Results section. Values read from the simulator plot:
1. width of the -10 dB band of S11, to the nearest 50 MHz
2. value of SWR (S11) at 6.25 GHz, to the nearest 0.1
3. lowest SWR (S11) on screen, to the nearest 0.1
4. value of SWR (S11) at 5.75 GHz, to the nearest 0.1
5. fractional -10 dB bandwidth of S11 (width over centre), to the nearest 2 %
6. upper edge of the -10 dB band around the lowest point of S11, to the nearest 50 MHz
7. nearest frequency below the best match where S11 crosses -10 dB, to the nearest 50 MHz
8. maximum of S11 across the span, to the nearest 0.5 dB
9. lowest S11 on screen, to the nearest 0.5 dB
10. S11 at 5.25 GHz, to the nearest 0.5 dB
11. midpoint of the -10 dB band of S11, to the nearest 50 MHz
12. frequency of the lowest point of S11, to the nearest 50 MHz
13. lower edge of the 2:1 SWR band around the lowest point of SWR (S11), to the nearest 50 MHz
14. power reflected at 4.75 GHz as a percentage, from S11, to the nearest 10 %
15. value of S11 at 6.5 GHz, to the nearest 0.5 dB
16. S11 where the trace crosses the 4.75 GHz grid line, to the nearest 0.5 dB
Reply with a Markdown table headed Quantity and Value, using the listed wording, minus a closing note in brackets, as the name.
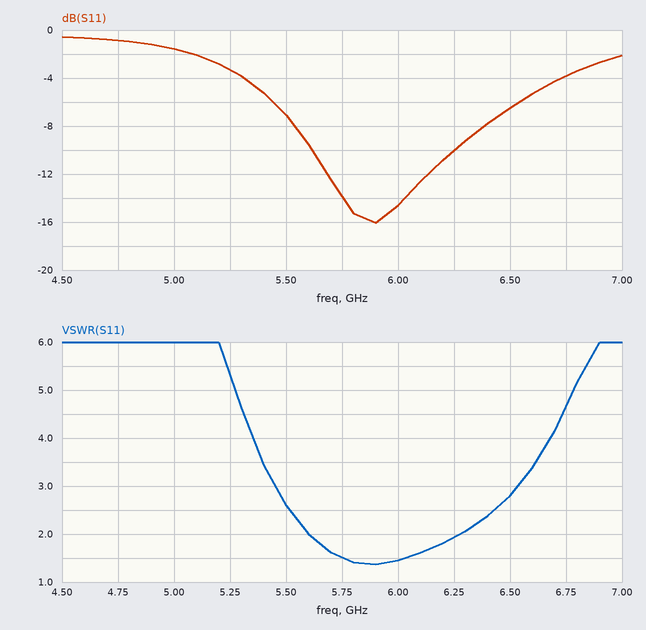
| Quantity | Value |
|---|---|
| width of the -10 dB band of S11, to the nearest 50 MHz | 650 MHz |
| value of SWR (S11) at 6.25 GHz, to the nearest 0.1 | 1.9 |
| lowest SWR (S11) on screen, to the nearest 0.1 | 1.4 |
| value of SWR (S11) at 5.75 GHz, to the nearest 0.1 | 1.5 |
| fractional -10 dB bandwidth of S11 (width over centre), to the nearest 2 % | 10 % |
| upper edge of the -10 dB band around the lowest point of S11, to the nearest 50 MHz | 6.25 GHz |
| nearest frequency below the best match where S11 crosses -10 dB, to the nearest 50 MHz | 5.60 GHz |
| maximum of S11 across the span, to the nearest 0.5 dB | -0.5 dB |
| lowest S11 on screen, to the nearest 0.5 dB | -16.0 dB |
| S11 at 5.25 GHz, to the nearest 0.5 dB | -3.5 dB |
| midpoint of the -10 dB band of S11, to the nearest 50 MHz | 5.95 GHz |
| frequency of the lowest point of S11, to the nearest 50 MHz | 5.90 GHz |
| lower edge of the 2:1 SWR band around the lowest point of SWR (S11), to the nearest 50 MHz | 5.60 GHz |
| power reflected at 4.75 GHz as a percentage, from S11, to the nearest 10 % | 80 % |
| value of S11 at 6.5 GHz, to the nearest 0.5 dB | -6.5 dB |
| S11 where the trace crosses the 4.75 GHz grid line, to the nearest 0.5 dB | -1.0 dB |
